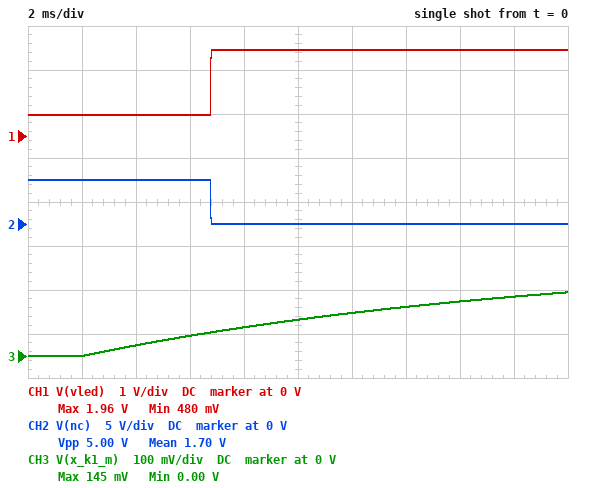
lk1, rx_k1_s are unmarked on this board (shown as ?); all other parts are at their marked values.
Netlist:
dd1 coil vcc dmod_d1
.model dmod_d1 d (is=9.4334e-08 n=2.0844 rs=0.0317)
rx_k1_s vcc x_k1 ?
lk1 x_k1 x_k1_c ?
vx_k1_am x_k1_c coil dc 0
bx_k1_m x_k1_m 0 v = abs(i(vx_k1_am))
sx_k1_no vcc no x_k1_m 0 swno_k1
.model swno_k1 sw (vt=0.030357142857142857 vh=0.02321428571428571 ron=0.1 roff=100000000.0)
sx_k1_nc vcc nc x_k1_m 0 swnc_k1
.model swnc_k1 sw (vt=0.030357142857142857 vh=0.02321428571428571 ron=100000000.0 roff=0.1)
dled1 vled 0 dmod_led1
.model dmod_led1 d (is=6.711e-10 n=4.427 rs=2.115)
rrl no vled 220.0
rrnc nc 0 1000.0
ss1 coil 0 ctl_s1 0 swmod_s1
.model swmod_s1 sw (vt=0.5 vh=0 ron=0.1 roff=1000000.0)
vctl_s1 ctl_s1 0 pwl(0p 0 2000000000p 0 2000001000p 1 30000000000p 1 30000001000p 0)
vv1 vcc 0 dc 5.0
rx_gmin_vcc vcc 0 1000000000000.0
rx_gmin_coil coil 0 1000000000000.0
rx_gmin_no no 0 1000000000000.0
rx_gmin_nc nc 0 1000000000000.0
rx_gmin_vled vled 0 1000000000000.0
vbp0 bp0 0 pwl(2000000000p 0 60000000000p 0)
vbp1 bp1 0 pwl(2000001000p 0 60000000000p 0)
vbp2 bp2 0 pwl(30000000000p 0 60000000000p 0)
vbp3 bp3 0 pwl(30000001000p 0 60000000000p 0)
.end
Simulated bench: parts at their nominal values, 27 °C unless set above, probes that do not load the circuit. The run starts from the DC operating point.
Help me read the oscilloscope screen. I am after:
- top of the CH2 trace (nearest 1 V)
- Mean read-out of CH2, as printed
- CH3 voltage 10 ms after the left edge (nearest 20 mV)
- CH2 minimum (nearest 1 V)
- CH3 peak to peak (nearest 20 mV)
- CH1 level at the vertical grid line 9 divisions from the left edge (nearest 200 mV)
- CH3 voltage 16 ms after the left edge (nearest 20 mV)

5 V
1.70 V
80 mV
0 V
140 mV
2.0 V
120 mV
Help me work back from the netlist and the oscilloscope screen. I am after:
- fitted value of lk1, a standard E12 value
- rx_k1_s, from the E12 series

390 mH
22 Ω
